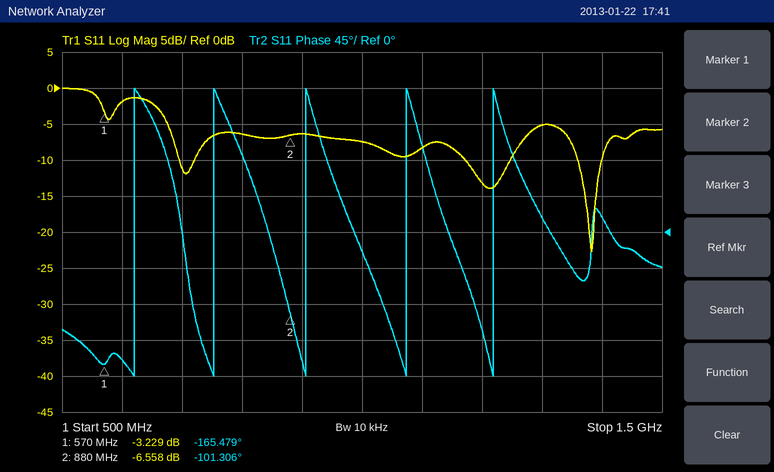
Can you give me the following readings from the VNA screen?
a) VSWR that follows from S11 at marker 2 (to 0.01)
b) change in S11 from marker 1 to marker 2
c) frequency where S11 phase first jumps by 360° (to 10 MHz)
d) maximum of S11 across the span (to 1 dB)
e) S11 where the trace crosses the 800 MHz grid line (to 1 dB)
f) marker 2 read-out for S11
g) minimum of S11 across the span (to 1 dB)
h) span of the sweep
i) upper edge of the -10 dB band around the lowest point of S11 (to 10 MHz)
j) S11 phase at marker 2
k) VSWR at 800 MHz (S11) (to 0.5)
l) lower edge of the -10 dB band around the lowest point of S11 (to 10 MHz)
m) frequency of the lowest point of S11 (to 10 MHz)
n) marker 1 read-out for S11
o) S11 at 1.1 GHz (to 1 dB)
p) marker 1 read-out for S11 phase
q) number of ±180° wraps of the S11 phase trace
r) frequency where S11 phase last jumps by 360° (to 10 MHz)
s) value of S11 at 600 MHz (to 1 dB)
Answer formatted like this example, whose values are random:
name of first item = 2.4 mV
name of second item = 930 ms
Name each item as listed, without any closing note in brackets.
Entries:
VSWR that follows from S11 at marker 2 = 2.77
change in S11 from marker 1 to marker 2 = -3.329 dB
frequency where S11 phase first jumps by 360° = 620 MHz
maximum of S11 across the span = 0 dB
S11 where the trace crosses the 800 MHz grid line = -6 dB
marker 2 read-out for S11 = -6.558 dB
minimum of S11 across the span = -23 dB
span of the sweep = 1 GHz
upper edge of the -10 dB band around the lowest point of S11 = 1.40 GHz
S11 phase at marker 2 = -101.306°
VSWR at 800 MHz (S11) = 3.0
lower edge of the -10 dB band around the lowest point of S11 = 1.36 GHz
frequency of the lowest point of S11 = 1.38 GHz
marker 1 read-out for S11 = -3.229 dB
S11 at 1.1 GHz = -8 dB
marker 1 read-out for S11 phase = -165.479°
number of ±180° wraps of the S11 phase trace = 5
frequency where S11 phase last jumps by 360° = 1.22 GHz
value of S11 at 600 MHz = -2 dB
